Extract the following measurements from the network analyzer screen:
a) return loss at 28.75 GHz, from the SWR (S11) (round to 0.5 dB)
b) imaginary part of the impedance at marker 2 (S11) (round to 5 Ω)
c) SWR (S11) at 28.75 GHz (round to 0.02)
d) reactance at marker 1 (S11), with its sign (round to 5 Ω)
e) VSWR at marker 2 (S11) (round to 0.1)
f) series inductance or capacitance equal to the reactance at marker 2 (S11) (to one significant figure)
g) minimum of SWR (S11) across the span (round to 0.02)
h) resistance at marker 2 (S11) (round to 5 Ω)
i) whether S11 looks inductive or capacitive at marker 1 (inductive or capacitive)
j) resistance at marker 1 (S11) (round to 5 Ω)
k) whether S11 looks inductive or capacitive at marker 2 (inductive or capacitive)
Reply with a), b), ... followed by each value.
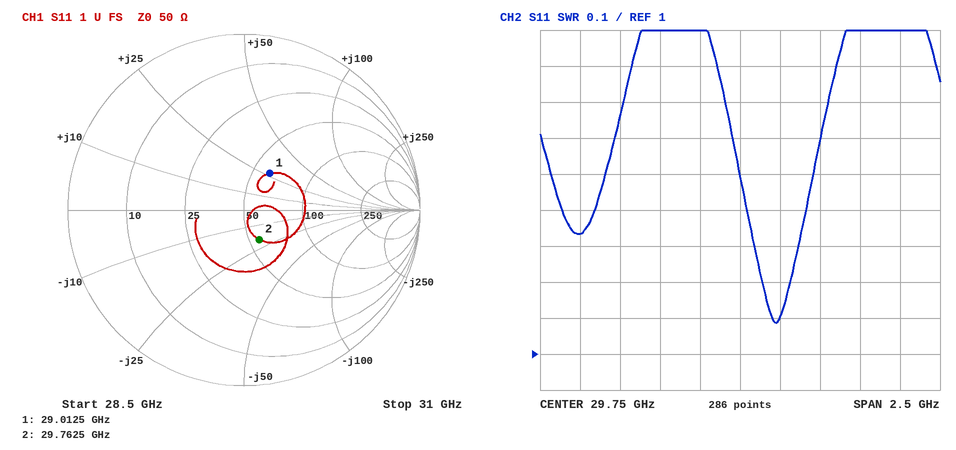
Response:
a) 17.0 dB
b) -20 Ω
c) 1.34
d) +25 Ω
e) 1.5
f) 300 fF
g) 1.08
h) 55 Ω
i) inductive
j) 60 Ω
k) capacitive
